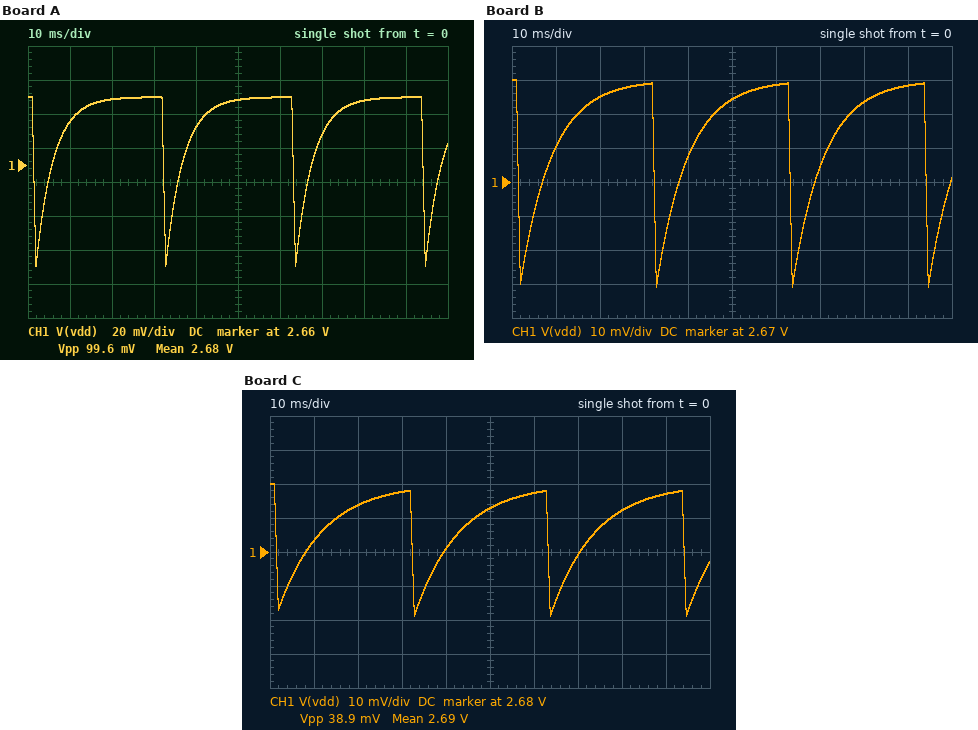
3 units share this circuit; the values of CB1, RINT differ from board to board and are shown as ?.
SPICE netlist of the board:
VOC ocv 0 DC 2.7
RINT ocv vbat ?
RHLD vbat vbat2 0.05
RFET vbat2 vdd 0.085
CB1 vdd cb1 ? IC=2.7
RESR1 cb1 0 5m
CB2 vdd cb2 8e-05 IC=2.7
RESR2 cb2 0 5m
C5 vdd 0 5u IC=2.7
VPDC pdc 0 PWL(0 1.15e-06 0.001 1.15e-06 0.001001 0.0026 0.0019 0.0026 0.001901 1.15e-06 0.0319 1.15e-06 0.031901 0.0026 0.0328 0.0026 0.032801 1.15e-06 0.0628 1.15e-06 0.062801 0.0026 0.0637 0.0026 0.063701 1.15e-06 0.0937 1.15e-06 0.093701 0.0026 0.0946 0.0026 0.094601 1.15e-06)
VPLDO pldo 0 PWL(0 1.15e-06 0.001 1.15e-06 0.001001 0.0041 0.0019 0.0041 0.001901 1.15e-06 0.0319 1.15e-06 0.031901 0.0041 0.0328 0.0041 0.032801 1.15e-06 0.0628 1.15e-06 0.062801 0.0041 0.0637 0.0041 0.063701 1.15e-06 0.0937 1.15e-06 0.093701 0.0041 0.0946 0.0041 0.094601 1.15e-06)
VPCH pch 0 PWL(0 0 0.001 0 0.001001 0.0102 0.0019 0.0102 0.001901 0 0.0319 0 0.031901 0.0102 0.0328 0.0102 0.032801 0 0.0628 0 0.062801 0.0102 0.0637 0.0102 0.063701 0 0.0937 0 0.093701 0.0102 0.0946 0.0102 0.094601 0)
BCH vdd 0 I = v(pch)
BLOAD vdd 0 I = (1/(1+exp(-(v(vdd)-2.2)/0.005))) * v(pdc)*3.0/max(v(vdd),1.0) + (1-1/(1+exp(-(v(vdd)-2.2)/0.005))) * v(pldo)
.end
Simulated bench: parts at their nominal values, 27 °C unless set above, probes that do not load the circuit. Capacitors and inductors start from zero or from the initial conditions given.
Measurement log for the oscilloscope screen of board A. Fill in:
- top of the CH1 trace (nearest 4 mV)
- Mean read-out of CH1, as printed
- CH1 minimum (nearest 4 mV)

2.700 V
2.68 V
2.600 V
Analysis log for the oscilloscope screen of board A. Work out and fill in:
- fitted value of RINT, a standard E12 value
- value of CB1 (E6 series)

39 Ω
22 µF
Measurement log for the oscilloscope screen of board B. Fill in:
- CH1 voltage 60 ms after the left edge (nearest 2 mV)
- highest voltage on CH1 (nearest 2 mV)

2.698 V
2.700 V
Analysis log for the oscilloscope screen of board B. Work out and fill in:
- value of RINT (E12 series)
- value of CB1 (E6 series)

39 Ω
100 µF
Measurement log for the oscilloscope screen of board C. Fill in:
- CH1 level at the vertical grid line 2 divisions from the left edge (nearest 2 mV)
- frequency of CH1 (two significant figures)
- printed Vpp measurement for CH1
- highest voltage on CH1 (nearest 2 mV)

2.694 V
32 Hz
38.9 mV
2.700 V
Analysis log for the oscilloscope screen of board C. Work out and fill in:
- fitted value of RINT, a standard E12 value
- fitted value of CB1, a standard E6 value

33 Ω
220 µF
